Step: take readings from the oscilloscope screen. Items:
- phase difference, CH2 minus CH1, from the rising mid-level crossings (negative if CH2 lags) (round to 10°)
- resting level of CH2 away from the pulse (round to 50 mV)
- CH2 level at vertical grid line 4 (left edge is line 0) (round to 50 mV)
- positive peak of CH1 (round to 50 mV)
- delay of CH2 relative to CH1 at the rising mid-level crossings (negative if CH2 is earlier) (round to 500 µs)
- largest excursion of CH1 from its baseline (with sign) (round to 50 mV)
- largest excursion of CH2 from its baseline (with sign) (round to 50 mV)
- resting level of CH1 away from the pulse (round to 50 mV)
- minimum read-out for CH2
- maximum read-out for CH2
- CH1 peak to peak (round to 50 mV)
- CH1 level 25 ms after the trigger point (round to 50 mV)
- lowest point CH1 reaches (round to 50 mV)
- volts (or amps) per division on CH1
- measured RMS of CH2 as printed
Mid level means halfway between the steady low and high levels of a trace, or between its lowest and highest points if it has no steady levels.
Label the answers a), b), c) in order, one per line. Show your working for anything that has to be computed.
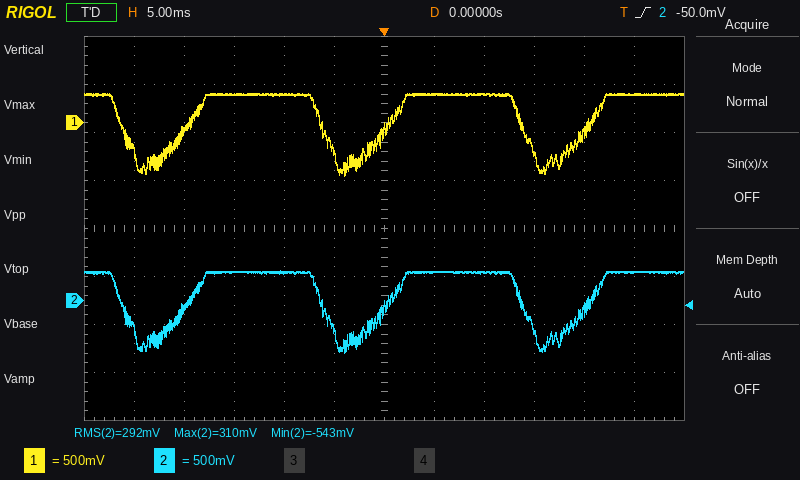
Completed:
a) 0°
b) 300 mV
c) 300 mV
d) 300 mV
e) 0.0 ms
f) -550 mV − (300 mV) = -850 mV
g) -850 mV
h) 300 mV
i) -543 mV
j) 310 mV
k) 300 mV − (-550 mV) = 850 mV
l) 300 mV
m) -550 mV
n) 500 mV
o) 292 mV
